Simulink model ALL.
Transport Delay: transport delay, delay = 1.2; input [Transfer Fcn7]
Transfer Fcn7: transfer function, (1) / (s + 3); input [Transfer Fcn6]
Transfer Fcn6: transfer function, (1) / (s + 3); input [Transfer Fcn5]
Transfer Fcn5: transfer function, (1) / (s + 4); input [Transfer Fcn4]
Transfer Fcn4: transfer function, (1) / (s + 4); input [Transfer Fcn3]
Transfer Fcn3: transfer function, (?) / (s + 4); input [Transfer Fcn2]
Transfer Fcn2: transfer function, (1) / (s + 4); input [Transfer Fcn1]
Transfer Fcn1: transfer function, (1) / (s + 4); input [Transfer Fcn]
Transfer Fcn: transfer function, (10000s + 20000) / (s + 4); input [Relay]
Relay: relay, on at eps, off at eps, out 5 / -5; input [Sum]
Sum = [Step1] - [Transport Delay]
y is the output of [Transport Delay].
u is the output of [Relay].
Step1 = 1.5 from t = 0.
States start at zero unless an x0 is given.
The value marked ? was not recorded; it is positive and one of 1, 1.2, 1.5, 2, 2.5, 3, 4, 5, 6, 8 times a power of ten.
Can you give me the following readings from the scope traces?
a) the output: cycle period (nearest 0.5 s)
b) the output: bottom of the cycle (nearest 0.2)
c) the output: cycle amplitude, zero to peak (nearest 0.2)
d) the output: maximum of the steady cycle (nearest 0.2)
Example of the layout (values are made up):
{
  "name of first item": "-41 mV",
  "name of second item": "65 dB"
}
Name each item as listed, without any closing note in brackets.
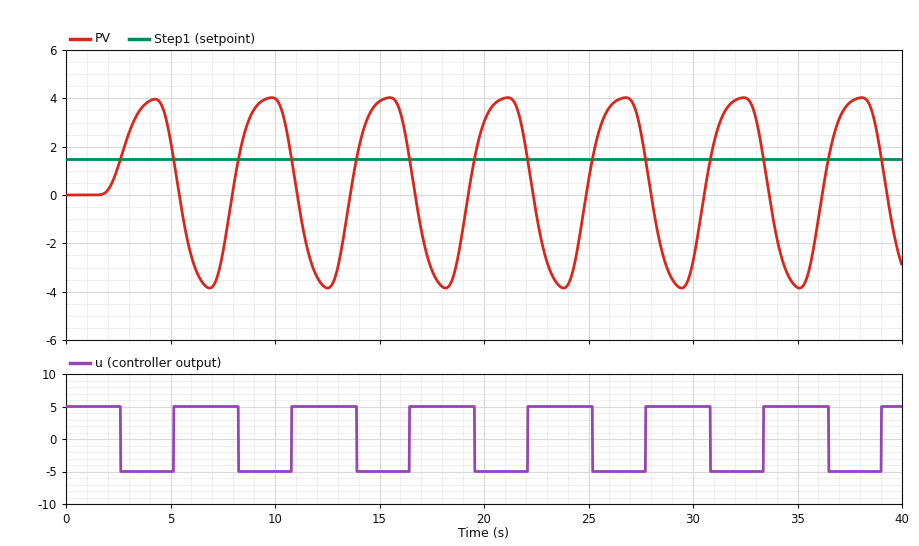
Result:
{
  "the output: cycle period": "5.5 s",
  "the output: bottom of the cycle": "-3.8",
  "the output: cycle amplitude, zero to peak": "4.0",
  "the output: maximum of the steady cycle": "4.0"
}
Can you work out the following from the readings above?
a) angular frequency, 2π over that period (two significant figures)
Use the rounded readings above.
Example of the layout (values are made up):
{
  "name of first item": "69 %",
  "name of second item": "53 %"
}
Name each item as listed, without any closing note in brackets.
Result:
{
  "angular frequency, 2π over that period": "1.1 rad/s"
}
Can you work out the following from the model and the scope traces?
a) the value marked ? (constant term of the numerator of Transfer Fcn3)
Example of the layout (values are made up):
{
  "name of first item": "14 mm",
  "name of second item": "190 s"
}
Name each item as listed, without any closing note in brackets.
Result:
{
  "the value marked ?": "1.5"
}
